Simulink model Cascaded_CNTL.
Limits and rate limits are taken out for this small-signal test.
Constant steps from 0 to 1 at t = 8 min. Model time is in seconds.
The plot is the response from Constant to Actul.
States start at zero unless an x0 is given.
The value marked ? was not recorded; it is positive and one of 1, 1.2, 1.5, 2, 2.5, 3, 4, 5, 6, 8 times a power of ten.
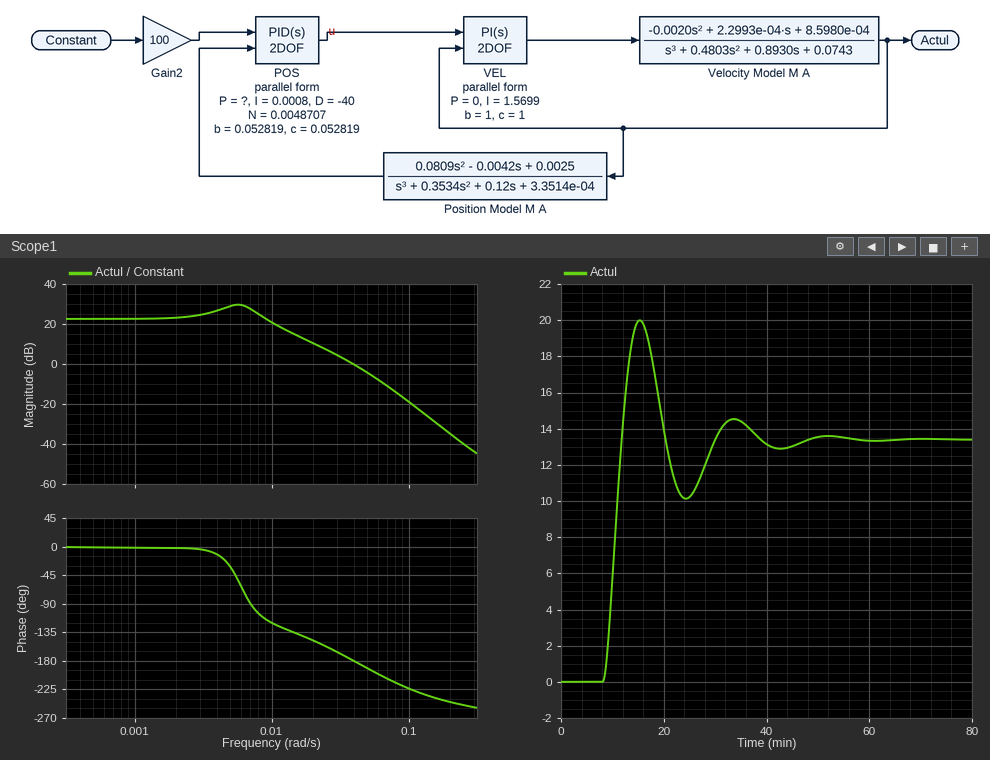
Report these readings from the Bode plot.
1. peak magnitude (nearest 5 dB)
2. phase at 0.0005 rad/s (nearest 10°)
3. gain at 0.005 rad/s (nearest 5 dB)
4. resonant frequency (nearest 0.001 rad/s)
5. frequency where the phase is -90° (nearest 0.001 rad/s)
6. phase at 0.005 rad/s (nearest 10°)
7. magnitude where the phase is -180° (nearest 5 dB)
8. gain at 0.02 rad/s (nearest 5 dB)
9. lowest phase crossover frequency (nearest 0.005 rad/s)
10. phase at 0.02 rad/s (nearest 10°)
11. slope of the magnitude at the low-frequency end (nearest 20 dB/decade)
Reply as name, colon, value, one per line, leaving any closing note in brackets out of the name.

peak magnitude: 30 dB
phase at 0.0005 rad/s: 0°
gain at 0.005 rad/s: 30 dB
resonant frequency: 0.006 rad/s
frequency where the phase is -90°: 0.007 rad/s
phase at 0.005 rad/s: -30°
magnitude where the phase is -180°: 0 dB
gain at 0.02 rad/s: 10 dB
lowest phase crossover frequency: 0.040 rad/s
phase at 0.02 rad/s: -150°
slope of the magnitude at the low-frequency end: 0 dB/decade
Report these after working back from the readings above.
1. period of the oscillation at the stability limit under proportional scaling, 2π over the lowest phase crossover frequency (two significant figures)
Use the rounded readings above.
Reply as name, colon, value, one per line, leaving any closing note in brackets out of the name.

period of the oscillation at the stability limit under proportional scaling, 2π over the lowest phase crossover frequency: 160 s
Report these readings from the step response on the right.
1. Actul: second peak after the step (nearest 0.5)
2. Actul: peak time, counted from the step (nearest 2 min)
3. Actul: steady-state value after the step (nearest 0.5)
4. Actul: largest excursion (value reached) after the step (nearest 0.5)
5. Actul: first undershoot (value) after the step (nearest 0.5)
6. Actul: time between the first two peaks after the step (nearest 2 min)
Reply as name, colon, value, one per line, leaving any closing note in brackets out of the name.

Actul: second peak after the step: 14.5
Actul: peak time, counted from the step: 8 min
Actul: steady-state value after the step: 13.5
Actul: largest excursion (value reached) after the step: 20.0
Actul: first undershoot (value) after the step: 10.0
Actul: time between the first two peaks after the step: 18 min
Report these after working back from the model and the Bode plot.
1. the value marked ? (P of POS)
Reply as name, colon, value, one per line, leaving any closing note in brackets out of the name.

the value marked ?: 0.2
